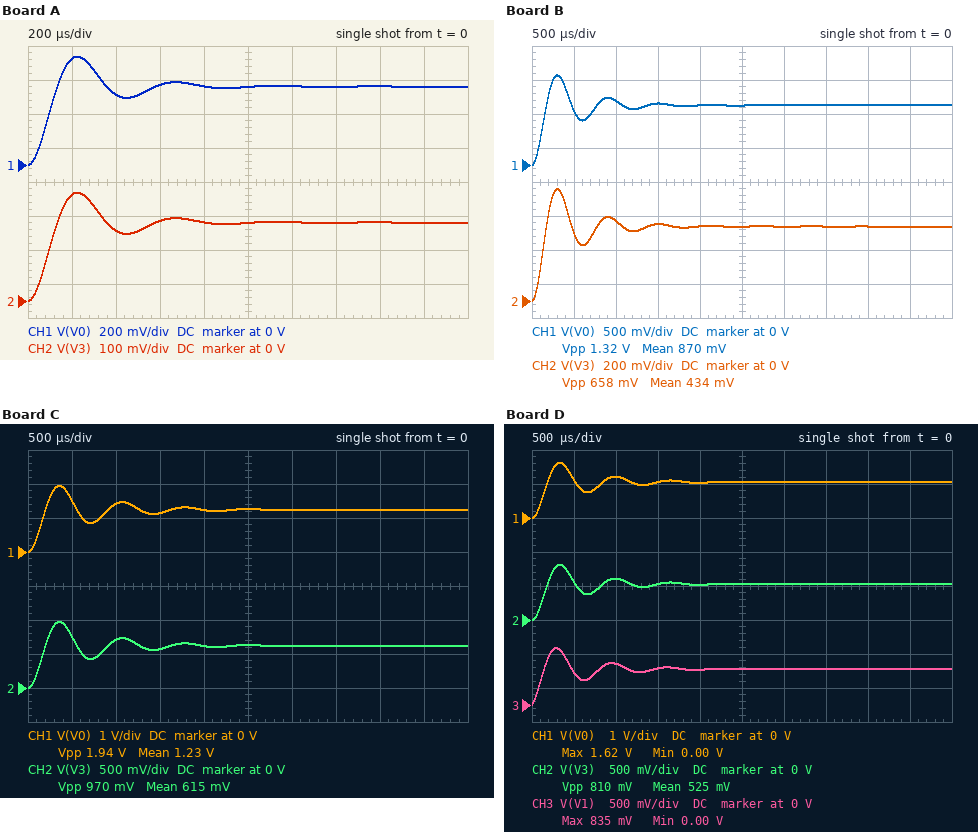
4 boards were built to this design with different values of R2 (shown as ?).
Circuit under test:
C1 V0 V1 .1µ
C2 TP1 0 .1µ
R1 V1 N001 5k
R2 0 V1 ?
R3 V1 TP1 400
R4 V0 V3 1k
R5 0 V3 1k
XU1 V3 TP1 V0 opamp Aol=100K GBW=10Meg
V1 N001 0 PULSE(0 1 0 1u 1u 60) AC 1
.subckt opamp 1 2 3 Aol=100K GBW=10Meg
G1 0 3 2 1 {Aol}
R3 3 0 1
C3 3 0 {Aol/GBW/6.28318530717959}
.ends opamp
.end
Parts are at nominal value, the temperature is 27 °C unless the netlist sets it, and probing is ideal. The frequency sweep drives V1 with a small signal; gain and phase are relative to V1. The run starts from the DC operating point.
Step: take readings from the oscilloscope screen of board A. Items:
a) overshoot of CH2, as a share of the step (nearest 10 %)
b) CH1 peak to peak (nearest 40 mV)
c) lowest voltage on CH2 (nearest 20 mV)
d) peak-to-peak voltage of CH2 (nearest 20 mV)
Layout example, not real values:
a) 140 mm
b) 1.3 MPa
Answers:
a) 40 %
b) 640 mV
c) 0 V
d) 320 mV
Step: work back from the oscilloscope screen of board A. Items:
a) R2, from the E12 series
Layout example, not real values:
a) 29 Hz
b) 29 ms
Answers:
a) 1.5 kΩ
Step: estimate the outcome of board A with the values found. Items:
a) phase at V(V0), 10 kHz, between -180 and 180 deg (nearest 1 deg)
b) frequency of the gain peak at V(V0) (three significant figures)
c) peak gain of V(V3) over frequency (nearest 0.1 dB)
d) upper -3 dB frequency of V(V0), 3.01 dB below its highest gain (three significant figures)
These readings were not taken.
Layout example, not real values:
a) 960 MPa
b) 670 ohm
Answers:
a) -172 deg
b) 2.13 kHz
c) -7.7 dB
d) 2.76 kHz
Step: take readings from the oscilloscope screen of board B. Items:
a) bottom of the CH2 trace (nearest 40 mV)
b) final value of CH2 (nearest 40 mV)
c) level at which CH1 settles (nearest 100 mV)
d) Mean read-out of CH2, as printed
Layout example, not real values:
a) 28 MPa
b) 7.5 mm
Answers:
a) 0 V
b) 440 mV
c) 900 mV
d) 434 mV
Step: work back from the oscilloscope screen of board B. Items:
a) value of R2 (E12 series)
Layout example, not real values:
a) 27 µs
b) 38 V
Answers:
a) 3.9 kΩ
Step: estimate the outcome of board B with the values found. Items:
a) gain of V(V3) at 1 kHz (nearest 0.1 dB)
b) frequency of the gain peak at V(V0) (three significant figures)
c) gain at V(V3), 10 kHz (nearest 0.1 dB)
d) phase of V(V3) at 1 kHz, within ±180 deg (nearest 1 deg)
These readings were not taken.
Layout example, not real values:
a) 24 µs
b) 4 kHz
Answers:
a) -4.1 dB
b) 1.62 kHz
c) -37.7 dB
d) -21 deg
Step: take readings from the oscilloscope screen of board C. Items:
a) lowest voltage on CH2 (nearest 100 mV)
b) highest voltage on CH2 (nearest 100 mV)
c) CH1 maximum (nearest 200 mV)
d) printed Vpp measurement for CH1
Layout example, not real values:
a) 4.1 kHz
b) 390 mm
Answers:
a) 0 V
b) 1.0 V
c) 2.0 V
d) 1.94 V
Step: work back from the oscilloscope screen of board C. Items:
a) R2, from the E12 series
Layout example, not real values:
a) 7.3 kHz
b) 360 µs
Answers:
a) 8.2 kΩ
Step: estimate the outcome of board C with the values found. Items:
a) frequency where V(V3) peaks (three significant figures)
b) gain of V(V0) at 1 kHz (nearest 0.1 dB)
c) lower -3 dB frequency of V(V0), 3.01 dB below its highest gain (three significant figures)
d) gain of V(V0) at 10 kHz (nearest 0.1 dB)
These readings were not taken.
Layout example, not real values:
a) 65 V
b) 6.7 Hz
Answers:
a) 1.38 kHz
b) 6.8 dB
c) 1.09 kHz
d) -31.8 dB
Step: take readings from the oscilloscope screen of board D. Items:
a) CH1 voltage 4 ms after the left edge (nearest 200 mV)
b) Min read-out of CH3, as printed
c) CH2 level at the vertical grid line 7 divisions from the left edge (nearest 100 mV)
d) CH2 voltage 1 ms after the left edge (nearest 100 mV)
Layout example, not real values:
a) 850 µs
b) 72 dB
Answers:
a) 1.0 V
b) 0.00 V
c) 500 mV
d) 600 mV
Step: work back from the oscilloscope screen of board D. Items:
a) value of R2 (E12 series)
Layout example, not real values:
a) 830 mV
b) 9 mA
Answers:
a) 5.6 kΩ
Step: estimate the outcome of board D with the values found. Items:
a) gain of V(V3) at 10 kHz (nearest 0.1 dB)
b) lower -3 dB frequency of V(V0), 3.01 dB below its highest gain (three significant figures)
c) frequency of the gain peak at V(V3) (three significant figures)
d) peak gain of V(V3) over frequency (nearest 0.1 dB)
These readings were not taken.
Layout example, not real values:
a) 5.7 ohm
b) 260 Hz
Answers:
a) -37.8 dB
b) 1.14 kHz
c) 1.49 kHz
d) 2.8 dB
